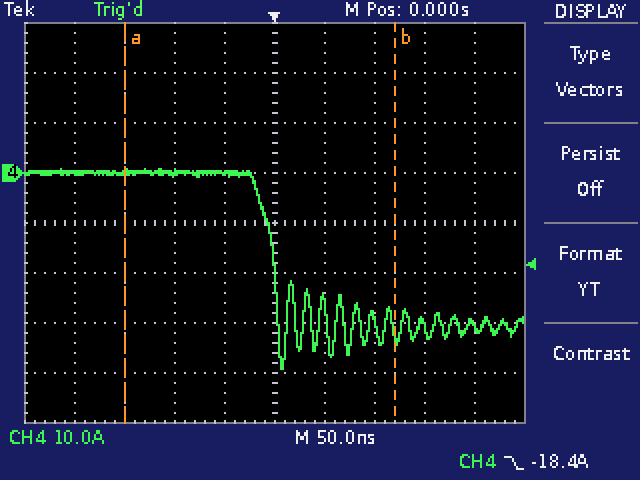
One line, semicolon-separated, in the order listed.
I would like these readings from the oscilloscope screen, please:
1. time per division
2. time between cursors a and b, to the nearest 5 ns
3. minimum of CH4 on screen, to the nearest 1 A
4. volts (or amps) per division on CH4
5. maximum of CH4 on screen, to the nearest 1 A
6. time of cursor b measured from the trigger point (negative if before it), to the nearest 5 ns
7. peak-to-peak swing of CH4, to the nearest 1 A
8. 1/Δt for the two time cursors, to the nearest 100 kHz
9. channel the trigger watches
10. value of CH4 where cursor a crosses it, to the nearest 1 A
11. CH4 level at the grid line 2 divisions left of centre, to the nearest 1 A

50 ns; 270 ns; -39 A; 10 A; 1 A; +120 ns; 40 A; 3.7 MHz; CH4; 0 A; 0 A
